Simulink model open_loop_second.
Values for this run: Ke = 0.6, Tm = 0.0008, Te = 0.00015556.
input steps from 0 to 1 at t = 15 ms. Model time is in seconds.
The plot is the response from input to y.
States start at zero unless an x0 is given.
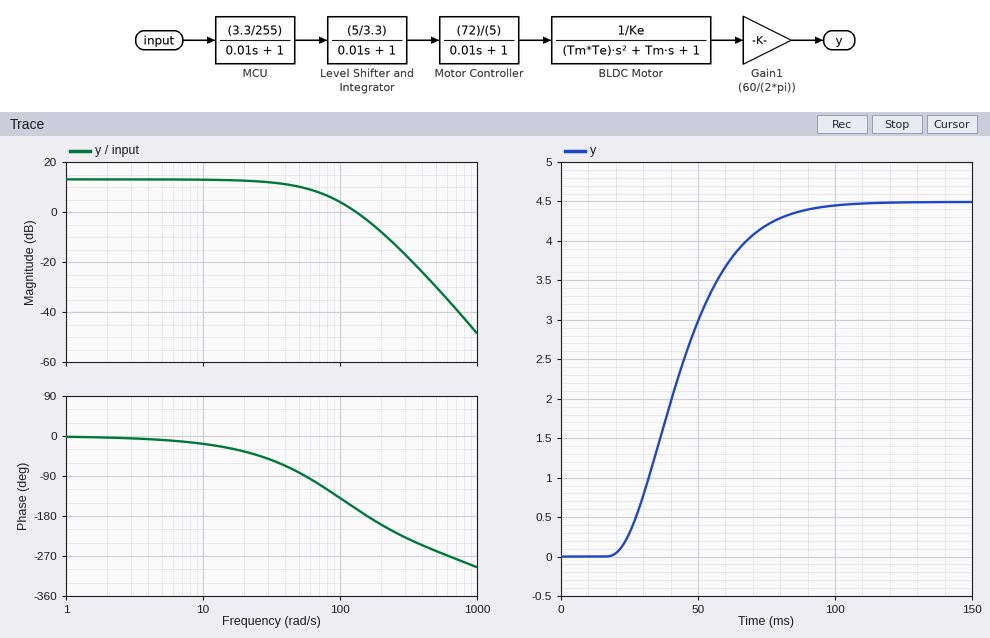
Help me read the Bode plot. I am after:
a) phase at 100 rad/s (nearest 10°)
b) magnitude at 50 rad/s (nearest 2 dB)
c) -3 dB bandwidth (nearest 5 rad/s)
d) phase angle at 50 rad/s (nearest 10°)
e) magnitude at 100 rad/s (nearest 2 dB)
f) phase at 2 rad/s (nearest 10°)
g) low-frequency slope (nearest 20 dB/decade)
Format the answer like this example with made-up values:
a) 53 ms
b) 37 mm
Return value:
a) -140°
b) 10 dB
c) 50 rad/s
d) -80°
e) 4 dB
f) 0°
g) 0 dB/decade
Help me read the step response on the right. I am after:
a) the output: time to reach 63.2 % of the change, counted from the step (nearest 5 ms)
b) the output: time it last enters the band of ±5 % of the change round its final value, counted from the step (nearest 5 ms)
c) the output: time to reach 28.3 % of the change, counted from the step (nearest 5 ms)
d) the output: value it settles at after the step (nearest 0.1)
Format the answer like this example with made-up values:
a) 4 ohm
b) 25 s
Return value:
a) 35 ms
b) 65 ms
c) 20 ms
d) 4.5
